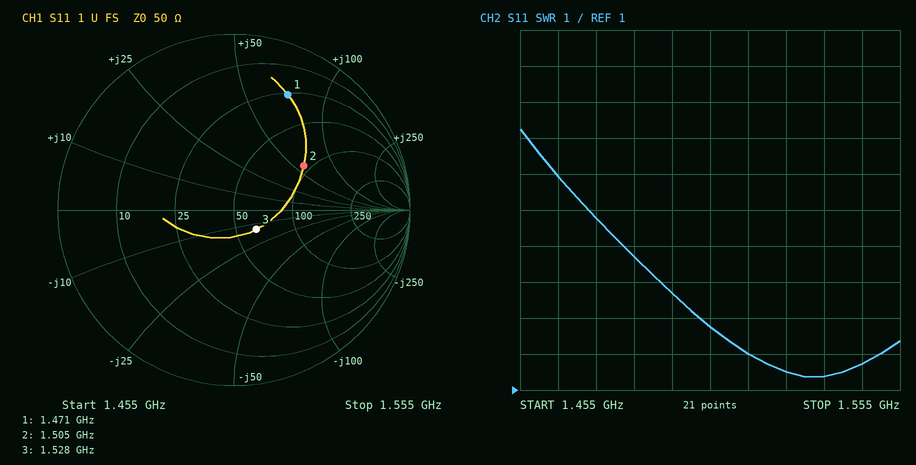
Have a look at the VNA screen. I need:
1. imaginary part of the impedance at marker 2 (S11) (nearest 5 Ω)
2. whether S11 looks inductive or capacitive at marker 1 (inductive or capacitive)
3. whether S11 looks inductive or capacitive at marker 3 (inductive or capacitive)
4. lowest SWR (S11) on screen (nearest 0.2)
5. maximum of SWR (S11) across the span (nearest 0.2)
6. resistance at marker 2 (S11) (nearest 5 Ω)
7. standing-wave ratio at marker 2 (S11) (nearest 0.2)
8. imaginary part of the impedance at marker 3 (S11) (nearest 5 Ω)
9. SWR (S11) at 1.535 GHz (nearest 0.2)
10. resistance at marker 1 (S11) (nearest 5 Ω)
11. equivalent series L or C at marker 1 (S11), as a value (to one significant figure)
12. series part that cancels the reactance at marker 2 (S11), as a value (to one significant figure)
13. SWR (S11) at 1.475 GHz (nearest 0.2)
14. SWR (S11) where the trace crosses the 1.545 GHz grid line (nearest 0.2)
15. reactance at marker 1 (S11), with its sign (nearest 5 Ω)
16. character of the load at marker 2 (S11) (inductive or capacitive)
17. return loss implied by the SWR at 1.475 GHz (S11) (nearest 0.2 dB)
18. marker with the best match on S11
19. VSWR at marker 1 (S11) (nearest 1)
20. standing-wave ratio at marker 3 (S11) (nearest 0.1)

+60 Ω
inductive
capacitive
1.4
8.2
90 Ω
2.8
-15 Ω
1.4
25 Ω
8 nH
2 pF
5.8
1.8
+70 Ω
inductive
3.0 dB
marker 3
6
1.4
